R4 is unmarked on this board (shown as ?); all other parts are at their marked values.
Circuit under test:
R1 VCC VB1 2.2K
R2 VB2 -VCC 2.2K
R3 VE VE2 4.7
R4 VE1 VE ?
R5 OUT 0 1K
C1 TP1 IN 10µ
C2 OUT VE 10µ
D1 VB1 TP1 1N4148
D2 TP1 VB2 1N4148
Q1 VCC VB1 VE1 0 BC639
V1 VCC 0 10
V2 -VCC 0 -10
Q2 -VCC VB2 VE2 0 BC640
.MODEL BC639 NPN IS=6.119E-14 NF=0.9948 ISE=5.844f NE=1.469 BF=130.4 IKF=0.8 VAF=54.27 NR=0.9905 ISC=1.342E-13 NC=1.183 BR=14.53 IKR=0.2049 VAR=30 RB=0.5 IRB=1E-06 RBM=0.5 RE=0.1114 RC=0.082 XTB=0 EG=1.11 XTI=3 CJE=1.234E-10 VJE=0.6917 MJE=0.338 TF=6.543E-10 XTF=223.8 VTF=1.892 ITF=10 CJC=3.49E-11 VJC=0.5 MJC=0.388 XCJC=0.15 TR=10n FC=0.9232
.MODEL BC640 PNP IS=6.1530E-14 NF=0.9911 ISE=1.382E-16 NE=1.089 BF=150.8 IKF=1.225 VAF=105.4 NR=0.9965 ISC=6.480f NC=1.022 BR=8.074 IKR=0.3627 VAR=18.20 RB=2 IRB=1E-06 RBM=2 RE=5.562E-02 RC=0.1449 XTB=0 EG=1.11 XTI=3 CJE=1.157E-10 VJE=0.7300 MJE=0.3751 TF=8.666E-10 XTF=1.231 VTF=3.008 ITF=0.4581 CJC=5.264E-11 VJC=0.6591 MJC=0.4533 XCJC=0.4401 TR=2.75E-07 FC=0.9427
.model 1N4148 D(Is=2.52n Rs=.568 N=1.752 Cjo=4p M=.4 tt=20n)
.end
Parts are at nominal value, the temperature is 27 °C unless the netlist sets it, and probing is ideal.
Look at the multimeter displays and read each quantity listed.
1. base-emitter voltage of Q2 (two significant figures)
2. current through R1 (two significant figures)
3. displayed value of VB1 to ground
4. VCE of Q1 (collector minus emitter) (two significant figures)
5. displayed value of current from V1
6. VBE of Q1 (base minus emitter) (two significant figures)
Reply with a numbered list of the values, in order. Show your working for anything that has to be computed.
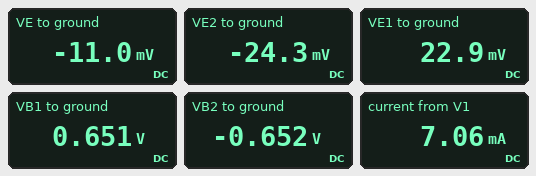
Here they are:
1. -652 mV - (-24.3 mV) = -630 mV
2. (10 V - 651 mV) / 2.2 kΩ = 4.2 mA
3. 0.651 V
4. 10 V - 22.9 mV = 10 V
5. 7.06 mA
6. 651 mV - 22.9 mV = 630 mV
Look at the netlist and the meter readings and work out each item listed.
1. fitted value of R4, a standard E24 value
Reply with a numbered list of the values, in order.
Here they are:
1. 12 Ω
